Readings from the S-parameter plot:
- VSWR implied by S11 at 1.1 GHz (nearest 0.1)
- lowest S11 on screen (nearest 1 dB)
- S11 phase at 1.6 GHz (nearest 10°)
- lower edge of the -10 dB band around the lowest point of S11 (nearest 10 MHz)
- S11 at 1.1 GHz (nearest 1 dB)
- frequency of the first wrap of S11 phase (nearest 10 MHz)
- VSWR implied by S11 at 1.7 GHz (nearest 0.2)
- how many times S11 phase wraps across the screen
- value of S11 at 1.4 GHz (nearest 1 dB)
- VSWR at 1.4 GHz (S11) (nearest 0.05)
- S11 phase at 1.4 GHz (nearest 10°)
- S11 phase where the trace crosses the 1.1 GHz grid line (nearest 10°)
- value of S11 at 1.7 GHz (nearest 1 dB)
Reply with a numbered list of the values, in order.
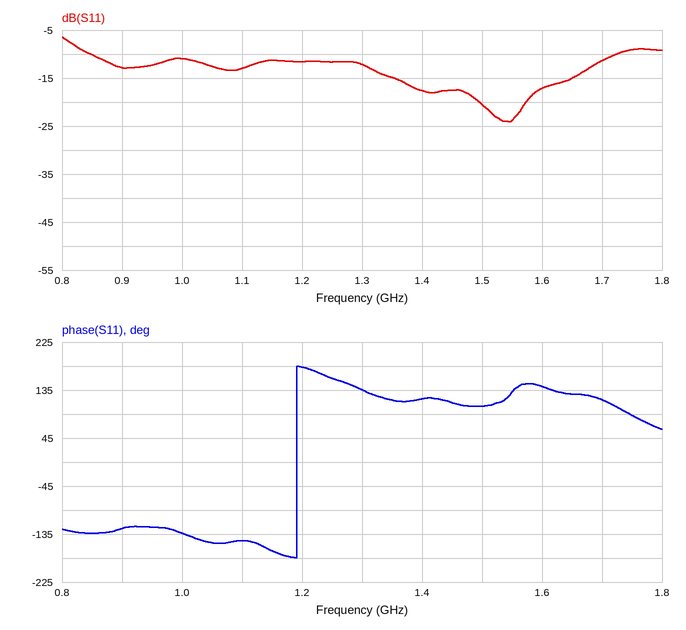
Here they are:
1. 1.6
2. -24 dB
3. 140°
4. 850 MHz
5. -13 dB
6. 1.19 GHz
7. 1.8
8. 1
9. -18 dB
10. 1.30
11. 120°
12. -150°
13. -11 dB
